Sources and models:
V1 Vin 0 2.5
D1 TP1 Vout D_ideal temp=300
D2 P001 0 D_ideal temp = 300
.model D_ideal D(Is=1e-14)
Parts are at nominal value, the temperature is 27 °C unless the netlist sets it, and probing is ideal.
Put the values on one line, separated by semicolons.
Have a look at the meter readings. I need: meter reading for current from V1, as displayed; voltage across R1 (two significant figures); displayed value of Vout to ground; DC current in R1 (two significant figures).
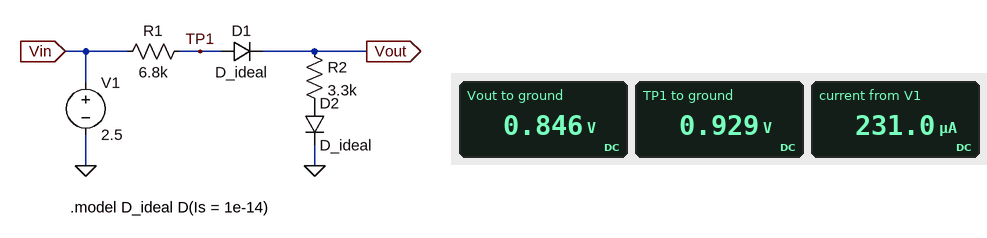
231.0 µA; 1.6 V; 0.846 V; 230 µA
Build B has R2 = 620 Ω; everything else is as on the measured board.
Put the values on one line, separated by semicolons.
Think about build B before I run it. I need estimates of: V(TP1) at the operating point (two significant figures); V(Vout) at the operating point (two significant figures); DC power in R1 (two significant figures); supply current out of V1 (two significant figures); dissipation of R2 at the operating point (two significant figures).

380 mV; 290 mV; 660 µW; 310 µA; 60 µW
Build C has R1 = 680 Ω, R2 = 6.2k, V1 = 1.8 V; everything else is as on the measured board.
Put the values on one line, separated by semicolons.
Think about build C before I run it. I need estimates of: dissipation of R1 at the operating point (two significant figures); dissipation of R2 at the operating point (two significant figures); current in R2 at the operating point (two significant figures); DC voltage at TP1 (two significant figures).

38 µW; 350 µW; 240 µA; 1.6 V
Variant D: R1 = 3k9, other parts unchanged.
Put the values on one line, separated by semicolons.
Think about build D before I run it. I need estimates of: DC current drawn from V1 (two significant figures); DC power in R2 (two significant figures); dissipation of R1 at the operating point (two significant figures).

320 µA; 340 µW; 400 µW
